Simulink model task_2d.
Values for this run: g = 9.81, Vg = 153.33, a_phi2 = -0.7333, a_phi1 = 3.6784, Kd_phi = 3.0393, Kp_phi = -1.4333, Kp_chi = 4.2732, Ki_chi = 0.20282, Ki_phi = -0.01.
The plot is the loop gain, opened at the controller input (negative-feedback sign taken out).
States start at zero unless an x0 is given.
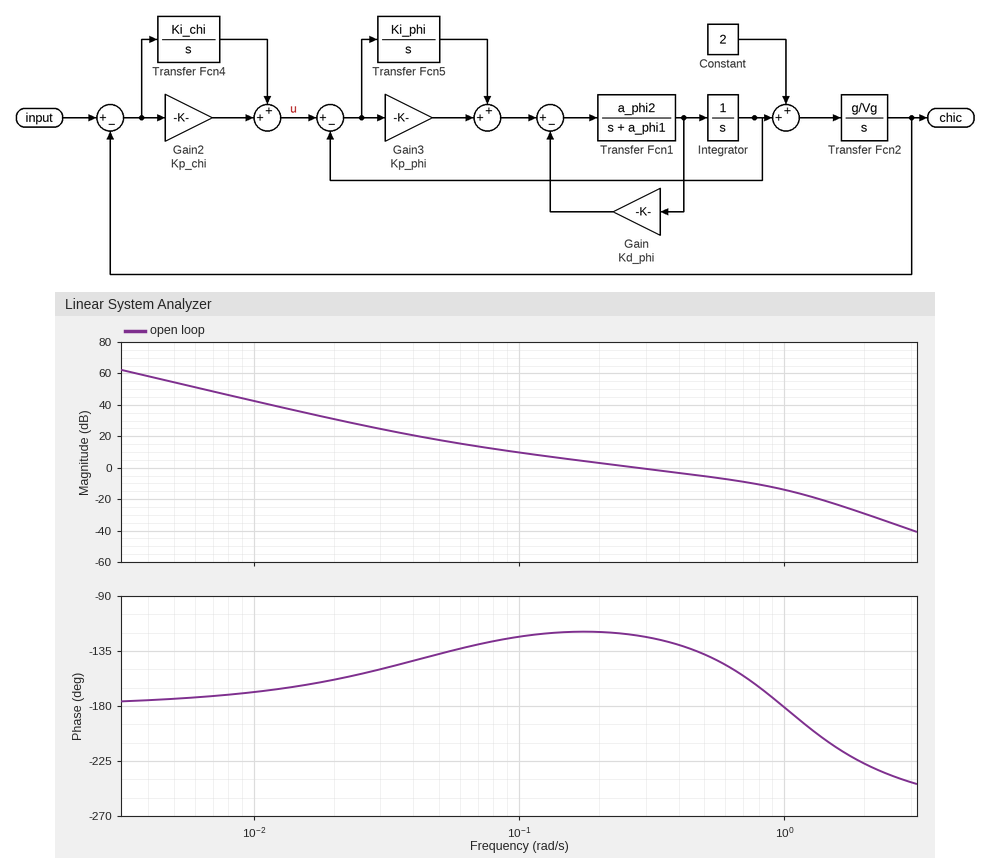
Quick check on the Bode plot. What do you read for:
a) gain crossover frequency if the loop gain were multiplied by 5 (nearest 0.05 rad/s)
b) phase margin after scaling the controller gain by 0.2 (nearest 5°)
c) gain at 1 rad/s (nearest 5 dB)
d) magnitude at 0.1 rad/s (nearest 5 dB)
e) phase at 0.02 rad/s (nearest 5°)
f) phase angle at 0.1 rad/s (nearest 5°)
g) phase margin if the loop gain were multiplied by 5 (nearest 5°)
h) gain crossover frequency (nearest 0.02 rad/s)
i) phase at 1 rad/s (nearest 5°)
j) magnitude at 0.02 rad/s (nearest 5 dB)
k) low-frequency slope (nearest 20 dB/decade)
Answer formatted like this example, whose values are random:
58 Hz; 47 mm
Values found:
1.00 rad/s; 50°; -15 dB; 10 dB; -160°; -125°; 0°; 0.28 rad/s; -180°; 30 dB; -40 dB/decade
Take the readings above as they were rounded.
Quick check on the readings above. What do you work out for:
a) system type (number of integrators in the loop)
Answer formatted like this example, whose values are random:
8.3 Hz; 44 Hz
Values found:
2
